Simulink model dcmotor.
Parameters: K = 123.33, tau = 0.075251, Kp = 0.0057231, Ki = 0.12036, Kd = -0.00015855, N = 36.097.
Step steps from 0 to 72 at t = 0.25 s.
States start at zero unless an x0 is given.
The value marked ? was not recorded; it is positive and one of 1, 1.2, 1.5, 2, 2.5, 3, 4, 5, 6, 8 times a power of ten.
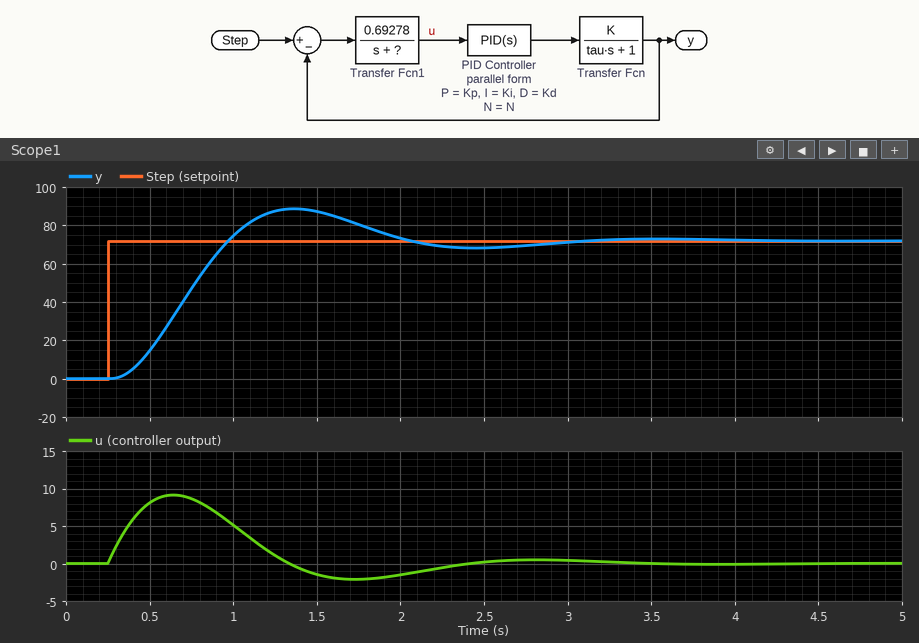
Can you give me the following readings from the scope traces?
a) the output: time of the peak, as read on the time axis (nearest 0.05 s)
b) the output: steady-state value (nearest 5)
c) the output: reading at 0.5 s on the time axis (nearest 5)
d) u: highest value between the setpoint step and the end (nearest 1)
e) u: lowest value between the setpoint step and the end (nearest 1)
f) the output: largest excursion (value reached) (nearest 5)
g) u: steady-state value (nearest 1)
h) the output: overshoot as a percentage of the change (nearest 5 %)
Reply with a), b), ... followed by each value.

a) 1.35 s
b) 70
c) 15
d) 9
e) -2
f) 90
g) 0
h) 25 %
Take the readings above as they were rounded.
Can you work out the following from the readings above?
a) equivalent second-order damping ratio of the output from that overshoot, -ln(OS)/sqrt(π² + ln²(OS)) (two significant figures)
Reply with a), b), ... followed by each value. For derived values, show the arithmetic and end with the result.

a) ln(0.25) = -1.386; 1.386 / sqrt(9.870 + 1.922) = 0.40
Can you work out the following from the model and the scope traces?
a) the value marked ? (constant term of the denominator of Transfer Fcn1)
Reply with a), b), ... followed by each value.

a) 3
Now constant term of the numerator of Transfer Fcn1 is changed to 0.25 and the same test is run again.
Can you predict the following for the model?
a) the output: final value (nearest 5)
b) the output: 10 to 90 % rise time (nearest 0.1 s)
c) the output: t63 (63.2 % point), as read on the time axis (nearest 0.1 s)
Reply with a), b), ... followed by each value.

a) 70
b) 1.2 s
c) 1.2 s
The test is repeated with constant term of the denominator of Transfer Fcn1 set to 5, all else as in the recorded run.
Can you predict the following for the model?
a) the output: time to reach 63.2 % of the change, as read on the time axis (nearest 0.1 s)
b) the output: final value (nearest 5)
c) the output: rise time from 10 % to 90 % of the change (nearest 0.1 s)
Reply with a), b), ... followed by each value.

a) 0.8 s
b) 70
c) 0.7 s
